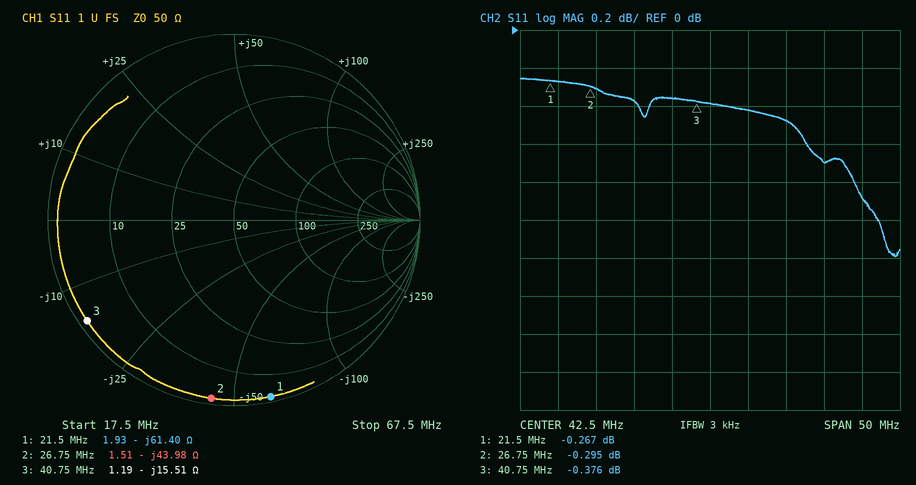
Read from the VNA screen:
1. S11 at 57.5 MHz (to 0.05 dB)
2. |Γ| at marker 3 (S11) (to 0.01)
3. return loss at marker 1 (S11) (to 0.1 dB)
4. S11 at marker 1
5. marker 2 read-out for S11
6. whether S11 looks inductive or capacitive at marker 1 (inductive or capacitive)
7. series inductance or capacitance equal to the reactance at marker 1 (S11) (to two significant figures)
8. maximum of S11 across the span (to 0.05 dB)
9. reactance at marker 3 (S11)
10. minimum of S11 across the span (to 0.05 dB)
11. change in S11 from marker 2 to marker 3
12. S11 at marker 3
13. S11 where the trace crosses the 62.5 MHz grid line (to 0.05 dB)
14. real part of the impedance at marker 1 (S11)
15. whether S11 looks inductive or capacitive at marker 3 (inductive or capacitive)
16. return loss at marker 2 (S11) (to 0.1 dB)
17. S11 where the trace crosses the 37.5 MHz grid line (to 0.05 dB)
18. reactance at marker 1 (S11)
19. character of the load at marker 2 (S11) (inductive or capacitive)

-0.70 dB
0.96
0.3 dB
-0.267 dB
-0.295 dB
capacitive
120 pF
-0.25 dB
-15.51 Ω
-1.20 dB
-0.081 dB
-0.376 dB
-0.90 dB
1.93 Ω
capacitive
0.3 dB
-0.35 dB
-61.40 Ω
capacitive
